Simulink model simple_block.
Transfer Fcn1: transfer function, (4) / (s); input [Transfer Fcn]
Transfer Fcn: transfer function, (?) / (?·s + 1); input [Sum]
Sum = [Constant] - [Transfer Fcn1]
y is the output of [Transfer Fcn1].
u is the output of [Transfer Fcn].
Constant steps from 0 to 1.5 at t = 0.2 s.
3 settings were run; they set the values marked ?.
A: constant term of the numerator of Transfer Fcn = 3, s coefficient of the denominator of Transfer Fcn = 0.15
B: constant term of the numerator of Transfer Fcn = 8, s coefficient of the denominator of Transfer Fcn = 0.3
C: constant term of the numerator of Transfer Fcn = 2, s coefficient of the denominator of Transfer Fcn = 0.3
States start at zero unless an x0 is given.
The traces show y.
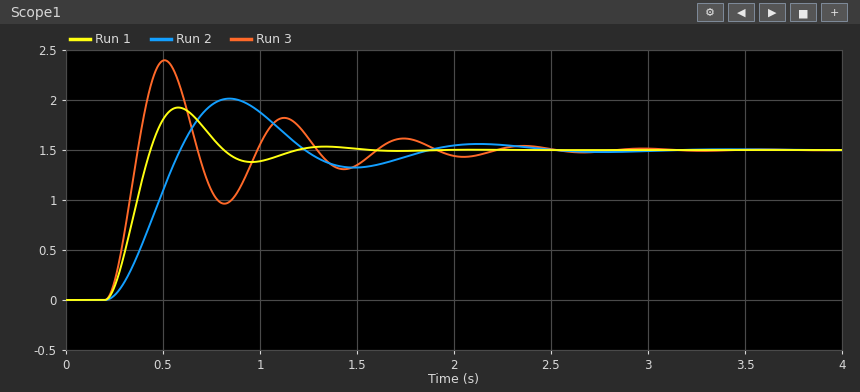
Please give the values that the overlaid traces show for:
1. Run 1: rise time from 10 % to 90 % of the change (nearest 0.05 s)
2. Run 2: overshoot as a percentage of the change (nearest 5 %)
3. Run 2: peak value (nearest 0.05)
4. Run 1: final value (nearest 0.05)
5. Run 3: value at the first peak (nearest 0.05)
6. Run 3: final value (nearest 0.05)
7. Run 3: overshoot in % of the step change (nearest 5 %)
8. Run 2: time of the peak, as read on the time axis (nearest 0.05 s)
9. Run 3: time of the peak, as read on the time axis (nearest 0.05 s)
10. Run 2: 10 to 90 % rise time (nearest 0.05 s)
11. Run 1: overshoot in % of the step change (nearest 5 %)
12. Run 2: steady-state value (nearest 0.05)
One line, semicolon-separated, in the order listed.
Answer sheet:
0.15 s; 35 %; 2.00; 1.50; 2.40; 1.50; 60 %; 0.85 s; 0.50 s; 0.25 s; 30 %; 1.50
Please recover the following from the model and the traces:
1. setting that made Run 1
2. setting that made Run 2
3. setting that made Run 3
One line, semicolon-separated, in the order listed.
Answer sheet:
A; C; B
